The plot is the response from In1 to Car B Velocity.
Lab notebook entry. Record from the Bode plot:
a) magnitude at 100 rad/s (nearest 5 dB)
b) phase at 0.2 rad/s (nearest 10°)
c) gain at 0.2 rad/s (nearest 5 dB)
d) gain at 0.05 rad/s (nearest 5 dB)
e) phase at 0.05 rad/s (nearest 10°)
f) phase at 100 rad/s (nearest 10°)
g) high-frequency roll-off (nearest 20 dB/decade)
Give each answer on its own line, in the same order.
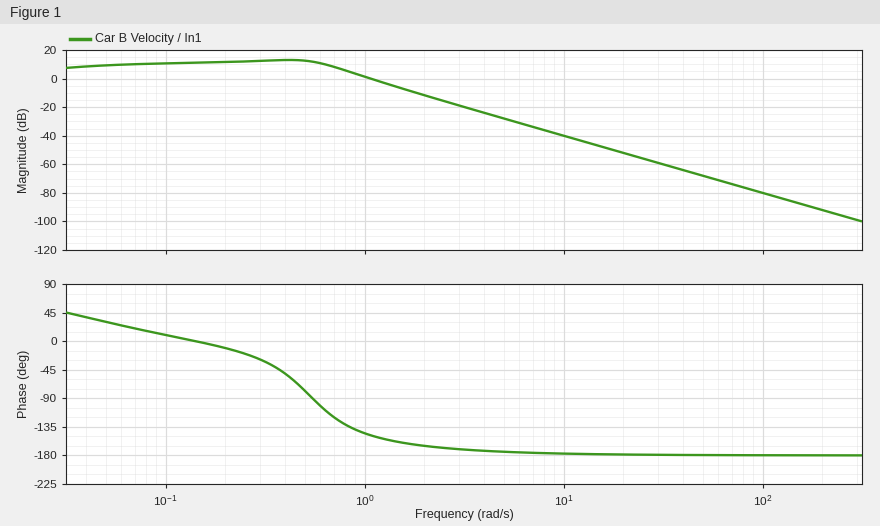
-80 dB
-10°
10 dB
10 dB
30°
-180°
-40 dB/decade
